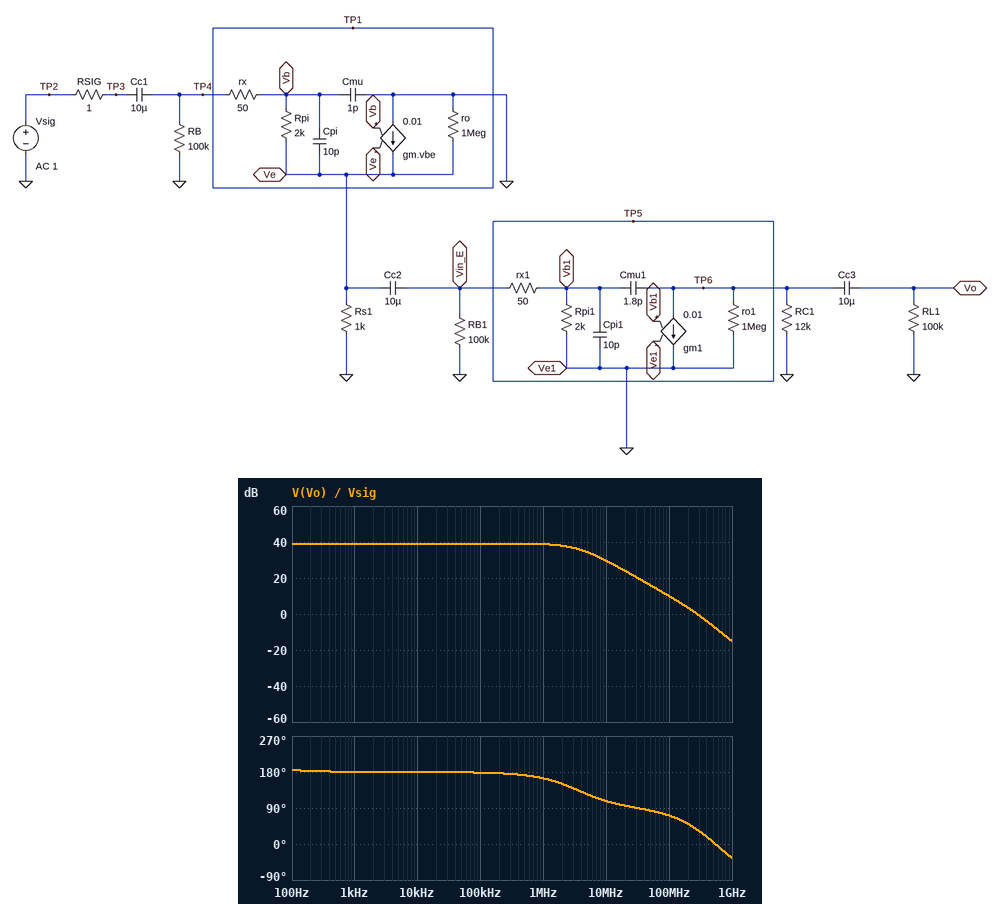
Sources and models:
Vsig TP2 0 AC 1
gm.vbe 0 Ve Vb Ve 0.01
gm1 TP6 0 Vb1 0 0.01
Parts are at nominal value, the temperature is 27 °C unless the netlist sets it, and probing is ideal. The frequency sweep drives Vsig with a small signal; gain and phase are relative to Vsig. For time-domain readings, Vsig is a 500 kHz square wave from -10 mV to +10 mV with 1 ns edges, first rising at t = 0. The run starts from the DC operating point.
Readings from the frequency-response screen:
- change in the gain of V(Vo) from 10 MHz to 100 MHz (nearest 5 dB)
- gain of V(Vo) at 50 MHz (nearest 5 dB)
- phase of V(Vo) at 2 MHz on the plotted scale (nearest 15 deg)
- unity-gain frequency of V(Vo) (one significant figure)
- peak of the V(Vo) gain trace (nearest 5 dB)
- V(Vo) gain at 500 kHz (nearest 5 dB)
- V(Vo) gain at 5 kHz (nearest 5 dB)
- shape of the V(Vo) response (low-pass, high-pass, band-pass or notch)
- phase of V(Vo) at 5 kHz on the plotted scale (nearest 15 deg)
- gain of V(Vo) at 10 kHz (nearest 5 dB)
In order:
-20 dB
15 dB
150 deg
300 MHz
40 dB
40 dB
40 dB
low-pass
180 deg
40 dB
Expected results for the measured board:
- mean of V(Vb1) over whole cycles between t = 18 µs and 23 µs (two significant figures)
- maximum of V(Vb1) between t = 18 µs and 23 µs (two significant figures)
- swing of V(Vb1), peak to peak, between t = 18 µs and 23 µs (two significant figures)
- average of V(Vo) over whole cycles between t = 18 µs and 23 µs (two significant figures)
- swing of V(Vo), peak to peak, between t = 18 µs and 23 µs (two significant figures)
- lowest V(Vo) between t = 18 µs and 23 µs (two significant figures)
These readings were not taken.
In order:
8.5 mV
17 mV
17 mV
-900 mV
1.8 V
-1.8 V
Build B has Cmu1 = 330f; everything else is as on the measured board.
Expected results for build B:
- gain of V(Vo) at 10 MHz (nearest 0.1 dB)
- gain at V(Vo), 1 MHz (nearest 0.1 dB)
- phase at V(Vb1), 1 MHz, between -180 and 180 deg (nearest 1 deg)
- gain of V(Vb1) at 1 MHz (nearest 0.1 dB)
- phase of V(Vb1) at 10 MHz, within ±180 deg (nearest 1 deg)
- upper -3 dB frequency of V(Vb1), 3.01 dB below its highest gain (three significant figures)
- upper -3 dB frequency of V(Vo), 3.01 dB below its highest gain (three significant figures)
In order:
37.9 dB
39.1 dB
-2 deg
-1.4 dB
-18 deg
21.0 MHz
17.6 MHz
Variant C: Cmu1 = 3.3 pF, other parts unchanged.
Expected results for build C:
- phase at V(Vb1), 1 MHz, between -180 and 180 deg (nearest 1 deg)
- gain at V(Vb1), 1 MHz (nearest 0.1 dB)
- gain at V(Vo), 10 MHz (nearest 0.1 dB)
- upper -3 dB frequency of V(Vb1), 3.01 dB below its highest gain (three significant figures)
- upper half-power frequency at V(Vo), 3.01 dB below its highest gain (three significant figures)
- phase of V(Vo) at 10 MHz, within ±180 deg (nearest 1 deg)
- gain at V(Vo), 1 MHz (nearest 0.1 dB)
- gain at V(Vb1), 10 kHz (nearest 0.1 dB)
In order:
-15 deg
-2.2 dB
24.7 dB
2.45 MHz
1.95 MHz
98 deg
38.1 dB
-1.4 dB
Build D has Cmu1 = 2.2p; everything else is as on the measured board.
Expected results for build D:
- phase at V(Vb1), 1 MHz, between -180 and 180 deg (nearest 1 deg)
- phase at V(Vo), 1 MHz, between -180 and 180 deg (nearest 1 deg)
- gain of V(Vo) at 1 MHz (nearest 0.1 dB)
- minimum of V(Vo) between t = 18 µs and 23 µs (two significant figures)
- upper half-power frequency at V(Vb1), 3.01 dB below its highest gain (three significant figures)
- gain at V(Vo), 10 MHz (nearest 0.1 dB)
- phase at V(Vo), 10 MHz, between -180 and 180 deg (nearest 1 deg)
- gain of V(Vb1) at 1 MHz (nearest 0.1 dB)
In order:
-11 deg
161 deg
38.6 dB
-1.8 V
3.64 MHz
28.0 dB
104 deg
-1.8 dB
